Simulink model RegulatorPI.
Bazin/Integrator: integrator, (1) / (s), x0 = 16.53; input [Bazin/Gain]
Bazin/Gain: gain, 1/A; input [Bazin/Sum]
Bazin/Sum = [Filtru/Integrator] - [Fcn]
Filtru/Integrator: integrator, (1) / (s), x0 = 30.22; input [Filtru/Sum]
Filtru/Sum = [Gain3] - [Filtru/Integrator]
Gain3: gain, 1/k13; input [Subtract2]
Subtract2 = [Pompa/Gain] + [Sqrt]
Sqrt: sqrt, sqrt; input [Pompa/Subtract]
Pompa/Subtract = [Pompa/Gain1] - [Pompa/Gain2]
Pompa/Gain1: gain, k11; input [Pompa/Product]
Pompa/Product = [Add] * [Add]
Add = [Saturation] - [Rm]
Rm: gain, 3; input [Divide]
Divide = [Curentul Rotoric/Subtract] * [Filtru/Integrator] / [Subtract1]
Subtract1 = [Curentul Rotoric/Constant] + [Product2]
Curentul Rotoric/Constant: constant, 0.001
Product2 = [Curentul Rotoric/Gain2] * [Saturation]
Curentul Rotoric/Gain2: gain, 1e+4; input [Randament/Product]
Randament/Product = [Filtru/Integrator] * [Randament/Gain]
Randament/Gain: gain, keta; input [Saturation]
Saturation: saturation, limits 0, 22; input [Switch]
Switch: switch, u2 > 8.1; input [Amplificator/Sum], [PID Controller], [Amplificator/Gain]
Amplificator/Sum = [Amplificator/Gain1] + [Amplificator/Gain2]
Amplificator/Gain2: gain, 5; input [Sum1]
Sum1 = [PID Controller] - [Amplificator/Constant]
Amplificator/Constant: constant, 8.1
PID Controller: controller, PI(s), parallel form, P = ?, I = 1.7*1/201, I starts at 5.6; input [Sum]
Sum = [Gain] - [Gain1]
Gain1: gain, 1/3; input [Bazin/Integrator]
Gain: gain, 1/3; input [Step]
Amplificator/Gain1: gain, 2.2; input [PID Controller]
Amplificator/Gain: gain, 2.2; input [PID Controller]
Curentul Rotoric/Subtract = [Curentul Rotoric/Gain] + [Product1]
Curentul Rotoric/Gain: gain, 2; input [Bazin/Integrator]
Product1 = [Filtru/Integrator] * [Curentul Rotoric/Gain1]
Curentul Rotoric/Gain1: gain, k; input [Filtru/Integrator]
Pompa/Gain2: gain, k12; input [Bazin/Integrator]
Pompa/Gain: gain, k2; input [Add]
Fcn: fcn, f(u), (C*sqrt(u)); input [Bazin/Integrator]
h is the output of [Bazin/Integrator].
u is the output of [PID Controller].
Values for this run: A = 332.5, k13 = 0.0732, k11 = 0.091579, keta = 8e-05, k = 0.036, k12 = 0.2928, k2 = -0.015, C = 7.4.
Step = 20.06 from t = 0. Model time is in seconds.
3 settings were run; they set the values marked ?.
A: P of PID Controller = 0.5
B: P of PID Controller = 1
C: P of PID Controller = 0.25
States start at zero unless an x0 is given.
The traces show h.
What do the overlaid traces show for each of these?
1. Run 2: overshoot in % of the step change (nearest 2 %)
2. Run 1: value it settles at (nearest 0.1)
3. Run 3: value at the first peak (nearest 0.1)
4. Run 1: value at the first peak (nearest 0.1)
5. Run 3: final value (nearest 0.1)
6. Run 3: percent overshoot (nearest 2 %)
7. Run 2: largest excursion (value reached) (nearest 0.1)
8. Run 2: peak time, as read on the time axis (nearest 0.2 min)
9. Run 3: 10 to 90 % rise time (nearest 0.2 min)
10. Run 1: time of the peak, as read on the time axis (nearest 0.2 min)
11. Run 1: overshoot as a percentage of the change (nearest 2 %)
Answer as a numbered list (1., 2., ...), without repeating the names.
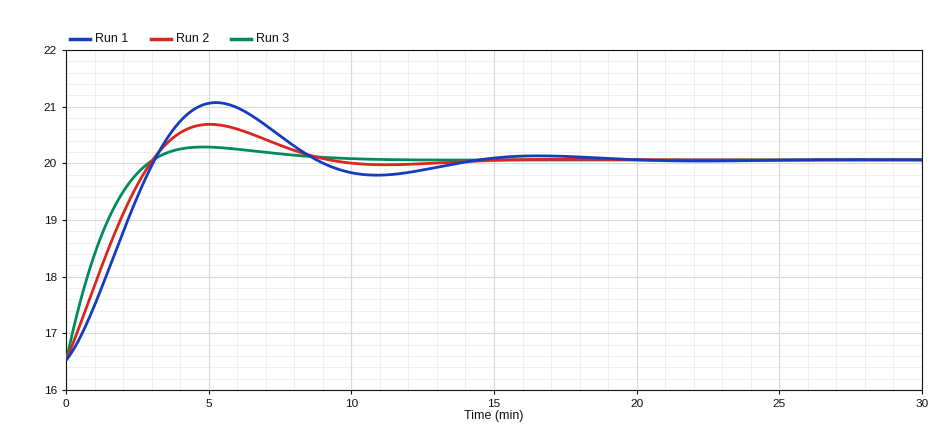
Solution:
1. 18 %
2. 20.1
3. 20.3
4. 21.1
5. 20.1
6. 6 %
7. 20.7
8. 5.0 min
9. 2.2 min
10. 5.2 min
11. 28 %
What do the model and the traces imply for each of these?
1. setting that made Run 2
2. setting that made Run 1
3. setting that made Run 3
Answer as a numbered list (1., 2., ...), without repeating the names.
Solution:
1. A
2. C
3. B
